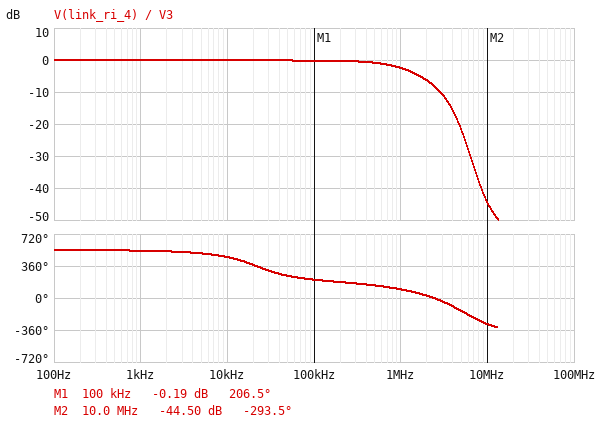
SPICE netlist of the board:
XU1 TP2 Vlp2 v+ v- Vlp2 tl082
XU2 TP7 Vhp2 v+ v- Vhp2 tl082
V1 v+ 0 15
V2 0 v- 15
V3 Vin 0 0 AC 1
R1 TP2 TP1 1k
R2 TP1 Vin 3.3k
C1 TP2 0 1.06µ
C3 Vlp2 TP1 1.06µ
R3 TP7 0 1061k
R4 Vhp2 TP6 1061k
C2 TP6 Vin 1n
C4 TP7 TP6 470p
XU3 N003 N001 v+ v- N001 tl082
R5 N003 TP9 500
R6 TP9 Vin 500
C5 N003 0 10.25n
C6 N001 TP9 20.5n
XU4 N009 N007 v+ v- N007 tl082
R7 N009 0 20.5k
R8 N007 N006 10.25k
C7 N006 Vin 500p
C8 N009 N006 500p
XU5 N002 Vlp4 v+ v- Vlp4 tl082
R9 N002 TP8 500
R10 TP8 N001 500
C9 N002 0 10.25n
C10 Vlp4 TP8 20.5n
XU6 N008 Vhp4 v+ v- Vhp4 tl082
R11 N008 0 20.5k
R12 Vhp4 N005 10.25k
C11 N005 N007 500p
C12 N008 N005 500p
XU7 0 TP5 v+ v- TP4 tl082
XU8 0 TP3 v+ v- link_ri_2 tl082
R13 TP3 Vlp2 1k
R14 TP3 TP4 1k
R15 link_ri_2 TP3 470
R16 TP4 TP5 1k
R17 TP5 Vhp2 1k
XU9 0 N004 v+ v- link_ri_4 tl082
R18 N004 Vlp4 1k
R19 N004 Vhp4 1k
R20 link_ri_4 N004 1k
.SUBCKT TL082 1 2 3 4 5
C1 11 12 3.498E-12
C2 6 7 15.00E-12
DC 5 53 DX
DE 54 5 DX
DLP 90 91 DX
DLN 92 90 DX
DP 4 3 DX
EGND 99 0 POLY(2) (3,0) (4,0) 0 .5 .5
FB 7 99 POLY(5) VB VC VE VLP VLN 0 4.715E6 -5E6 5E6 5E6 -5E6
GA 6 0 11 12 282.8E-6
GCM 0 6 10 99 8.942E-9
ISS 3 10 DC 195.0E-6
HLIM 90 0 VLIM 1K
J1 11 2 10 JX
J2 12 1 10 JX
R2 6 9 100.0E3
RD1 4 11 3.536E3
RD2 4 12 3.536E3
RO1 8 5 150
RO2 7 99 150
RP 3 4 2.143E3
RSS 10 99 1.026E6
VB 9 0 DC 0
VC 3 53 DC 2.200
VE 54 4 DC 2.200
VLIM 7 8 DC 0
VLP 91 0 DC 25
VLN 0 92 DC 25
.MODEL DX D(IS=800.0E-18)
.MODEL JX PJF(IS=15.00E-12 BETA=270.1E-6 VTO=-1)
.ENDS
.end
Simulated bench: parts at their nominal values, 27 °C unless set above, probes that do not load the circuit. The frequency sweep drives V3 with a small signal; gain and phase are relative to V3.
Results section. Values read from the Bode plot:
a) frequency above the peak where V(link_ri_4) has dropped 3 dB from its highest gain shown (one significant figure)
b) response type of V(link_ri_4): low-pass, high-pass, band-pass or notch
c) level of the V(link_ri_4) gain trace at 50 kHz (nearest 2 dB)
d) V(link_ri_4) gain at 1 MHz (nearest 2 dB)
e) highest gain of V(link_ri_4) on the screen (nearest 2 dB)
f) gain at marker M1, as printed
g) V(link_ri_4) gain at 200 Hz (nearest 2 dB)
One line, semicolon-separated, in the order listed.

1 MHz; low-pass; 0 dB; -2 dB; 0 dB; -0.19 dB; 0 dB
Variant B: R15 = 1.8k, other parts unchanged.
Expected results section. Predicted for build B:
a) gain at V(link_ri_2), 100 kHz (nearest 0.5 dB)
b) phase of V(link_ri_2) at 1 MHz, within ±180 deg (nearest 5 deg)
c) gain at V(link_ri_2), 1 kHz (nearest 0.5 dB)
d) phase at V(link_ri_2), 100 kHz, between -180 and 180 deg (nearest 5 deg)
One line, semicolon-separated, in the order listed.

5.0 dB; -120 deg; 4.5 dB; -15 deg
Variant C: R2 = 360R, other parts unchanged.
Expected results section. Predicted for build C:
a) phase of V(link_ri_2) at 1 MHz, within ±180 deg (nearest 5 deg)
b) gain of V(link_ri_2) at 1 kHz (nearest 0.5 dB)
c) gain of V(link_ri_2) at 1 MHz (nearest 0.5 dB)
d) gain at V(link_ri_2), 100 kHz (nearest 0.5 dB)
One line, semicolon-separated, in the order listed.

-105 deg; -6.5 dB; -8.0 dB; -6.5 dB
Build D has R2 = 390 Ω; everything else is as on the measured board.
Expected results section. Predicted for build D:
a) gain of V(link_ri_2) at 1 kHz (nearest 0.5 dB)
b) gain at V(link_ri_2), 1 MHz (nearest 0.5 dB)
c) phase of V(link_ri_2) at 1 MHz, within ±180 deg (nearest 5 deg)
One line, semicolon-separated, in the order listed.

-6.5 dB; -8.0 dB; -105 deg
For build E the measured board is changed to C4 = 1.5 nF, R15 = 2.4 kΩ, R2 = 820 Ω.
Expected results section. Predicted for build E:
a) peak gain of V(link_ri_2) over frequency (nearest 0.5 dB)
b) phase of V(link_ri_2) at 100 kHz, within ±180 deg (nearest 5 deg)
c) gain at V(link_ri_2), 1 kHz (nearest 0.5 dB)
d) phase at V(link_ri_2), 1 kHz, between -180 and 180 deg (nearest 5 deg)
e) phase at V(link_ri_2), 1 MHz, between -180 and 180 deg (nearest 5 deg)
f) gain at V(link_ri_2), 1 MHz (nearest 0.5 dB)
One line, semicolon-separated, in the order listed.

8.5 dB; -15 deg; 7.5 dB; 15 deg; -130 deg; 1.0 dB
